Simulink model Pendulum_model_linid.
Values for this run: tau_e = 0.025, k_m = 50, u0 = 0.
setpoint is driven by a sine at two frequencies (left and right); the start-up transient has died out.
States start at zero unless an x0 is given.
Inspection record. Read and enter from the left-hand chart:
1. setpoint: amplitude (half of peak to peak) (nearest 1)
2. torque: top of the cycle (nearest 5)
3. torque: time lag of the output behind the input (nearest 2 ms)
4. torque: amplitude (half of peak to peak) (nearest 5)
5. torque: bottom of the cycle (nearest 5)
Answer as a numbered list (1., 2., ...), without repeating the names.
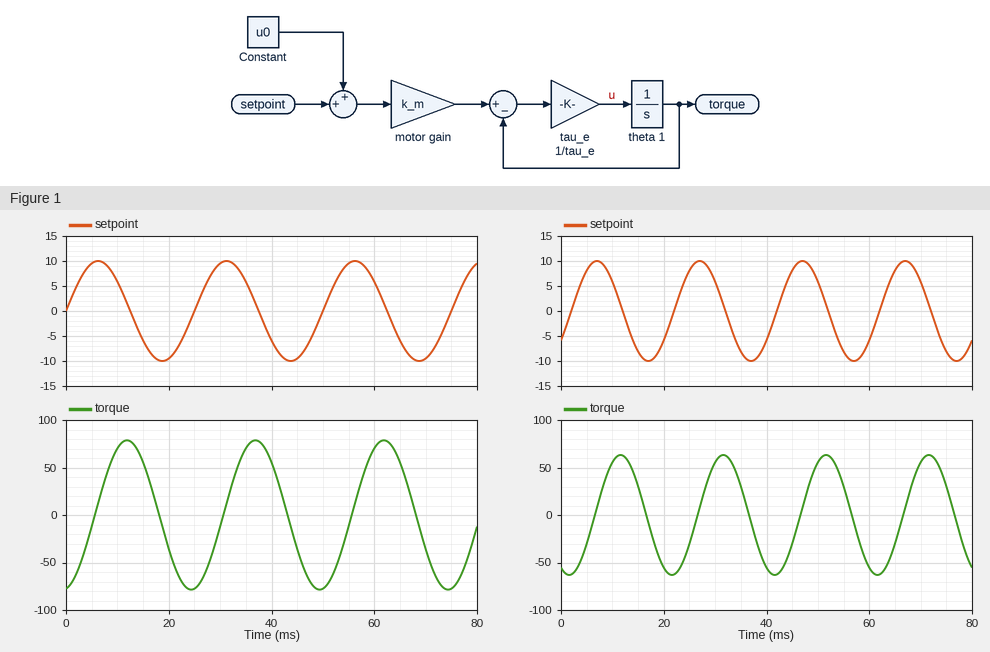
1. 10
2. 80
3. 6 ms
4. 80
5. -80
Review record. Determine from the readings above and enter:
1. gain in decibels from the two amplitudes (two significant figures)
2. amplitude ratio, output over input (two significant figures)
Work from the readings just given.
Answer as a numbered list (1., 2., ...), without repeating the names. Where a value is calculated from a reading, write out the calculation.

1. 20 log10(80 / 10) = 18 dB
2. 80 / 10 = 8.0
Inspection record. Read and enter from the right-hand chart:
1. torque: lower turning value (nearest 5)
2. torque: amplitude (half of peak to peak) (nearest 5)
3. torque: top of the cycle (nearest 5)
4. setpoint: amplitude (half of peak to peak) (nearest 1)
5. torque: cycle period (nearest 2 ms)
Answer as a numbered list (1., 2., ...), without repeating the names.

1. -65
2. 65
3. 65
4. 10
5. 20 ms
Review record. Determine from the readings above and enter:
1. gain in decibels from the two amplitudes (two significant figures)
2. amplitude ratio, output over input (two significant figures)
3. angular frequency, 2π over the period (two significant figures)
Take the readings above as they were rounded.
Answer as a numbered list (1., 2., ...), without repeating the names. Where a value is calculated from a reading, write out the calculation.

1. 20 log10(65 / 10) = 16 dB
2. 65 / 10 = 6.5
3. 2π / 20 = 0.31 rad/ms
